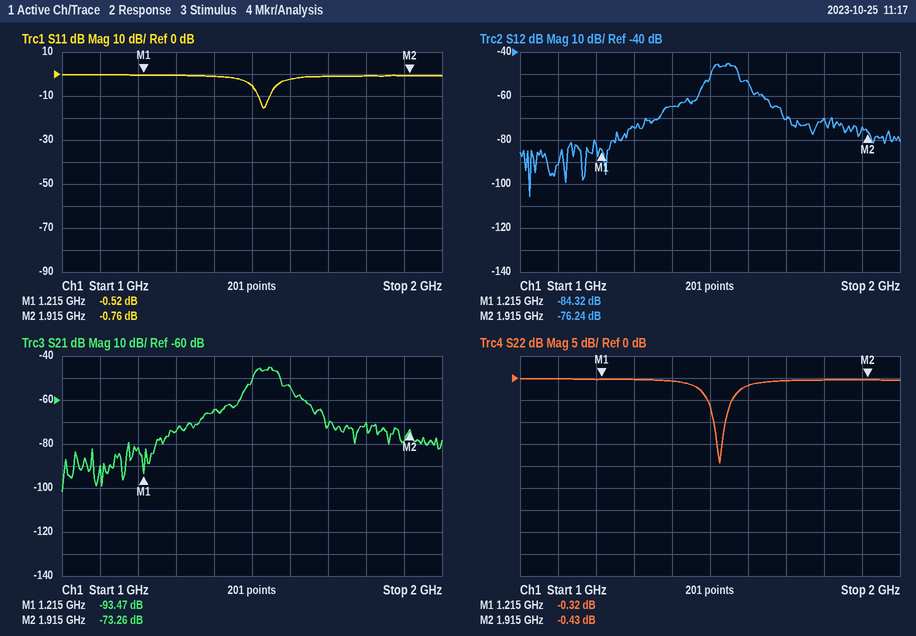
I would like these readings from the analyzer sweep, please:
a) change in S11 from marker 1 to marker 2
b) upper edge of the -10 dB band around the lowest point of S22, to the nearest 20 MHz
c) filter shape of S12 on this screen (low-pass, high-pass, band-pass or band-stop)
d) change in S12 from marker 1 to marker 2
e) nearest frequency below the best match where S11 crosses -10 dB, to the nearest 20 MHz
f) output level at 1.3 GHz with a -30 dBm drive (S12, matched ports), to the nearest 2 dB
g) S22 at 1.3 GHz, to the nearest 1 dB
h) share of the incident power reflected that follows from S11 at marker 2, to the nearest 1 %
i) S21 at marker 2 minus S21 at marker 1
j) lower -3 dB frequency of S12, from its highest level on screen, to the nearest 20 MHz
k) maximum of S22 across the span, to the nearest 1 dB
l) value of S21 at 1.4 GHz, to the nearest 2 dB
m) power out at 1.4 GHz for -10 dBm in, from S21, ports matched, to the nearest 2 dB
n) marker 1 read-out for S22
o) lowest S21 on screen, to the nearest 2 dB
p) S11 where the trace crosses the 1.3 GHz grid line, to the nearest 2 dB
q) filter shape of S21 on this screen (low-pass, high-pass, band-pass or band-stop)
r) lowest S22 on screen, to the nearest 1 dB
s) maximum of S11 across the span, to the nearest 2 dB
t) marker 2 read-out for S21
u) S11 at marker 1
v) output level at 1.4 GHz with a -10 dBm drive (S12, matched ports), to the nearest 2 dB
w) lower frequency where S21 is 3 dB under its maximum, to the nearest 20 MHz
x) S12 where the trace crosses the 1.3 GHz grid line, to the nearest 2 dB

-0.24 dB
1.54 GHz
band-pass
8.08 dB
1.52 GHz
-104 dBm
0 dB
84 %
20.21 dB
1.50 GHz
0 dB
-64 dB
-74 dBm
-0.32 dB
-102 dB
0 dB
band-pass
-19 dB
0 dB
-73.26 dB
-0.52 dB
-74 dBm
1.50 GHz
-74 dB
